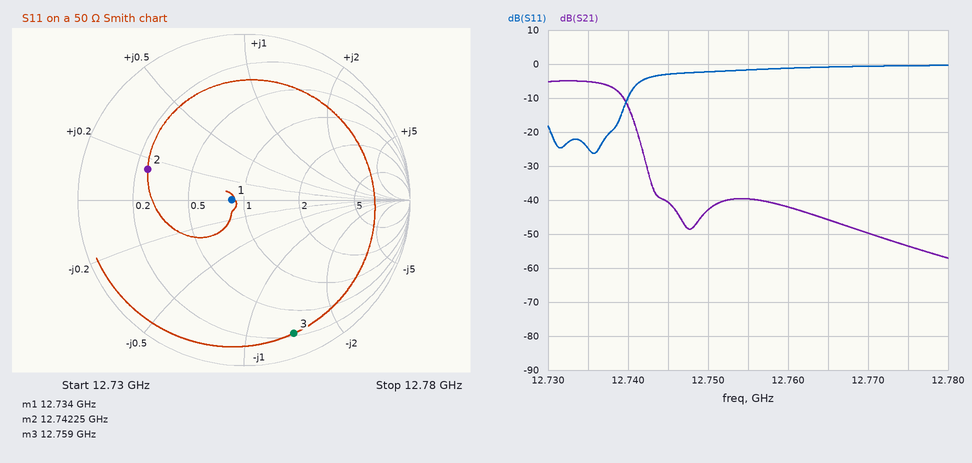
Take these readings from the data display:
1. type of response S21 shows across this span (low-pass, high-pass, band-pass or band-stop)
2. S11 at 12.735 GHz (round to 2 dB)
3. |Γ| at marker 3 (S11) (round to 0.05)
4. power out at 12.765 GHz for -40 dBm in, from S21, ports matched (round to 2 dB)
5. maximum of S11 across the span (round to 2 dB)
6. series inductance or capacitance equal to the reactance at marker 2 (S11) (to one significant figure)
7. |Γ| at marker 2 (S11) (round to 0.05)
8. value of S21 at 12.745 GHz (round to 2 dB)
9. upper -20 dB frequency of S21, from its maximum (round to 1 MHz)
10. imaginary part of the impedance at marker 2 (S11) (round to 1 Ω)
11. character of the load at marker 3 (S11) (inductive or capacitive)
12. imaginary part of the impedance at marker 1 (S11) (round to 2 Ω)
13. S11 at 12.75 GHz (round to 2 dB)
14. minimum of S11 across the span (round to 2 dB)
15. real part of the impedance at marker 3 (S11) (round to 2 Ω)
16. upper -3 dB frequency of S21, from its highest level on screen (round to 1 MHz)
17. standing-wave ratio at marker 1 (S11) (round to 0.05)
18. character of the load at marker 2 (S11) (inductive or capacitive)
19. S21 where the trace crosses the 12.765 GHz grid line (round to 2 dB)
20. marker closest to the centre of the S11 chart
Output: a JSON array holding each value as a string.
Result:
["low-pass", "-24 dB", "0.85", "-86 dBm", "0 dB", "90 pH", "0.60", "-40 dB", "12.742 GHz", "+7 Ω", "capacitive", "0 Ω", "-2 dB", "-26 dB", "12 Ω", "12.739 GHz", "1.15", "inductive", "-46 dB", "marker 1"]
